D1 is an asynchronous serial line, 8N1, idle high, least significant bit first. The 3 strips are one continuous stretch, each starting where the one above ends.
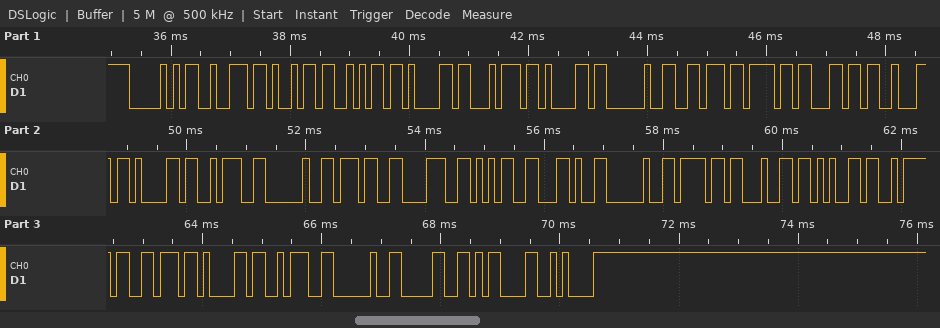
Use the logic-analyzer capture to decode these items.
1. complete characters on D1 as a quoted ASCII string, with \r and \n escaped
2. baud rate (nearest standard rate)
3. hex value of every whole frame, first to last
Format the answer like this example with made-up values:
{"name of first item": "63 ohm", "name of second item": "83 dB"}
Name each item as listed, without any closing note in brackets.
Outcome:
{"complete characters on D1 as a quoted ASCII string, with \\r and \\n escaped": "\"Prijata volba: 785, odezva: 0\\r\\n\"", "baud rate": "9600 baud", "hex value of every whole frame, first to last": "0x50 0x72 0x69 0x6A 0x61 0x74 0x61 0x20 0x76 0x6F 0x6C 0x62 0x61 0x3A 0x20 0x37 0x38 0x35 0x2C 0x20 0x6F 0x64 0x65 0x7A 0x76 0x61 0x3A 0x20 0x30 0x0D 0x0A"}
